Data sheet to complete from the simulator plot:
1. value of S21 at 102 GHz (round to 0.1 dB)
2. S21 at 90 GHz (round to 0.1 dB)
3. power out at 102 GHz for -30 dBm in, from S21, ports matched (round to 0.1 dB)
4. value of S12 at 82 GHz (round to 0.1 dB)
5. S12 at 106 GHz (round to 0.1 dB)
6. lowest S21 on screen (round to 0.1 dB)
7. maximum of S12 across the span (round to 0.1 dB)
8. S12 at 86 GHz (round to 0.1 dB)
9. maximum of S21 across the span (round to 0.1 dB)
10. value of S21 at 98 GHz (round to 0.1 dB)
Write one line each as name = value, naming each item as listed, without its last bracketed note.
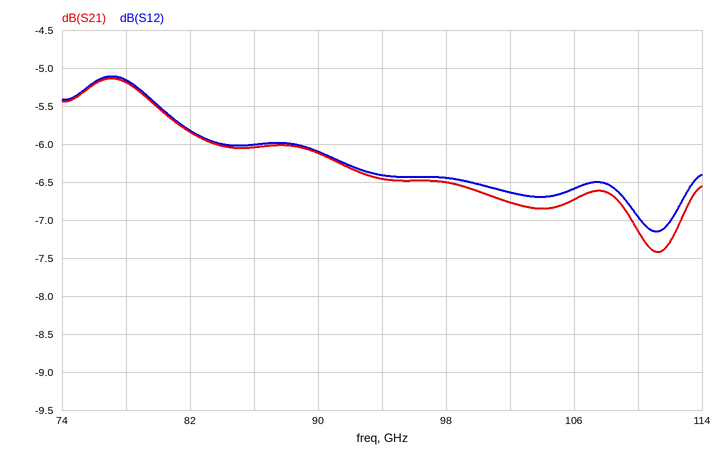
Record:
value of S21 at 102 GHz = -6.8 dB
S21 at 90 GHz = -6.1 dB
power out at 102 GHz for -30 dBm in, from S21, ports matched = -36.8 dBm
value of S12 at 82 GHz = -5.8 dB
S12 at 106 GHz = -6.6 dB
lowest S21 on screen = -7.4 dB
maximum of S12 across the span = -5.1 dB
S12 at 86 GHz = -6.0 dB
maximum of S21 across the span = -5.1 dB
value of S21 at 98 GHz = -6.5 dB
